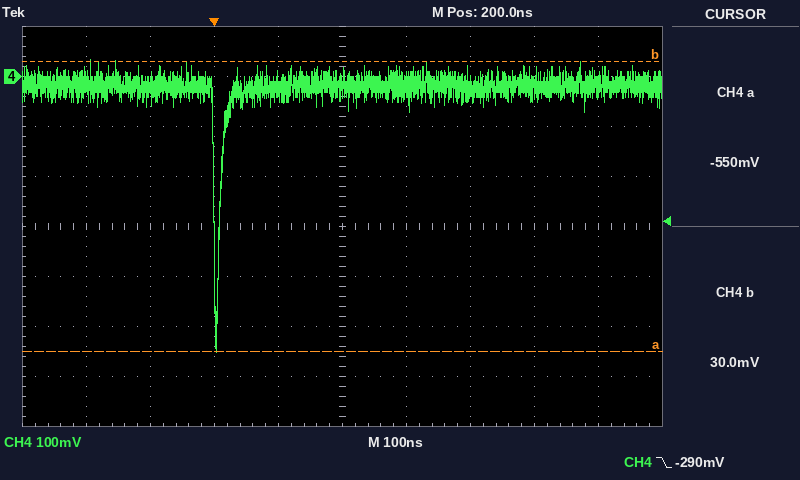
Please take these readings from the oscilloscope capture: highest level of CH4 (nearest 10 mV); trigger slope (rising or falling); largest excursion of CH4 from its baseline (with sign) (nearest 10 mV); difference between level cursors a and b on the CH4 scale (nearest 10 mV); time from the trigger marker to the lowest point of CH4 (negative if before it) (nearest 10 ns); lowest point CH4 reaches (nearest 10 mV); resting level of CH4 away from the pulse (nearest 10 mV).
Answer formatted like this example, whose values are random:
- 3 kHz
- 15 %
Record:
- 30 mV
- falling
- -530 mV
- 580 mV
- 0 ns
- -550 mV
- -20 mV
